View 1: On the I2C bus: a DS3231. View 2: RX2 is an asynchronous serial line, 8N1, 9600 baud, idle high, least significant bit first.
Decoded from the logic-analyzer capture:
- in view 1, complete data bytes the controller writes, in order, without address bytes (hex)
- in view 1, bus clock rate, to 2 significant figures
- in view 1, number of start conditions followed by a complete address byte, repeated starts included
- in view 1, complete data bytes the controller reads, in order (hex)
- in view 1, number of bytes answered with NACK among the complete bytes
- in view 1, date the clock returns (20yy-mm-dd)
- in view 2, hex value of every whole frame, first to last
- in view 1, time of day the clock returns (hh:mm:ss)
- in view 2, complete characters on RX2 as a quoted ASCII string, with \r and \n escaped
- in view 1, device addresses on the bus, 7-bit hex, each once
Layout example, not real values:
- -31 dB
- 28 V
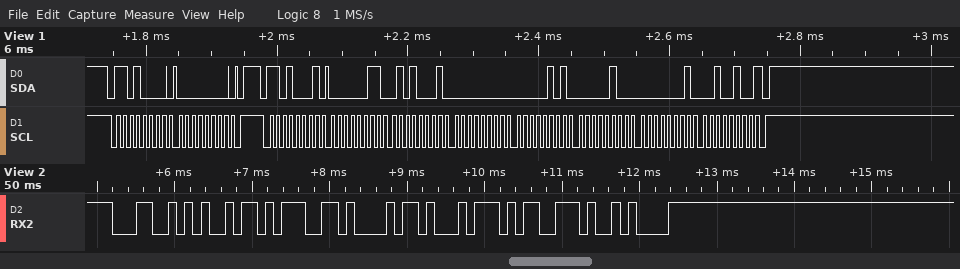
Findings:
- 00
- 100 kHz
- 2
- 03 51 00 05 04 01 24
- 1
- 2024-01-04
- 4C 69 67 68 74 73 0A
- 00:51:03
- "Lights\n"
- 0x68
